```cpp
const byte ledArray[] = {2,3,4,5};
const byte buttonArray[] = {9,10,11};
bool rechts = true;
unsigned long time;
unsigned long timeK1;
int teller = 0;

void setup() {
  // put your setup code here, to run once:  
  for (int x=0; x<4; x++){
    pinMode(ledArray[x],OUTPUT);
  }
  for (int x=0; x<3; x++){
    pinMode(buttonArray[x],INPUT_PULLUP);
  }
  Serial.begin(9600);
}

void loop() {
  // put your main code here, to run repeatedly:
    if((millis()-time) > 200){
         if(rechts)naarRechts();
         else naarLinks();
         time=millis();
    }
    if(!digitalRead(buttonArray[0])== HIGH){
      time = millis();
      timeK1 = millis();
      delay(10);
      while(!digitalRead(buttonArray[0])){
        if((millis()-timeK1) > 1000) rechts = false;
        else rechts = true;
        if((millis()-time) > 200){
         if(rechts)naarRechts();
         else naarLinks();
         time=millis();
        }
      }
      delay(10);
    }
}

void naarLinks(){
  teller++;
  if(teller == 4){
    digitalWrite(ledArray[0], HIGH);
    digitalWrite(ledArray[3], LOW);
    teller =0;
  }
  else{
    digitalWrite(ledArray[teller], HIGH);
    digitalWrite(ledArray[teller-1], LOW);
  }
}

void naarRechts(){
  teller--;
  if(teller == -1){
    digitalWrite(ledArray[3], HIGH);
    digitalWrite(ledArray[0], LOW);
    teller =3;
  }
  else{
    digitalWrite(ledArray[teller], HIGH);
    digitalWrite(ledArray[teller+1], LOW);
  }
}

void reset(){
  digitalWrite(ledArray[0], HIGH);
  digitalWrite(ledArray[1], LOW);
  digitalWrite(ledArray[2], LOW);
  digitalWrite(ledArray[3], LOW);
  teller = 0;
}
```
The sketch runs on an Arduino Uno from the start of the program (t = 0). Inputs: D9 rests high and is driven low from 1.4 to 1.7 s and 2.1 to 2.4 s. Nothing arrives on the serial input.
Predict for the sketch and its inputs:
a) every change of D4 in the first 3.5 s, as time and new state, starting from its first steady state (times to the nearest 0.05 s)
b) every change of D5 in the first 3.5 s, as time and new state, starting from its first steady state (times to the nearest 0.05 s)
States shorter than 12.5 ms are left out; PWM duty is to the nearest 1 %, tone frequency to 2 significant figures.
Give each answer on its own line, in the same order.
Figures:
0 s low; 0.4 s high; 0.6 s low; 1.2 s high; 1.6 s low; 2.3 s high; 2.5 s low; 3.1 s high; 3.3 s low
0 s low; 0.2 s high; 0.4 s low; 1 s high; 1.2 s low; 2 s high; 2.3 s low; 2.9 s high; 3.1 s low
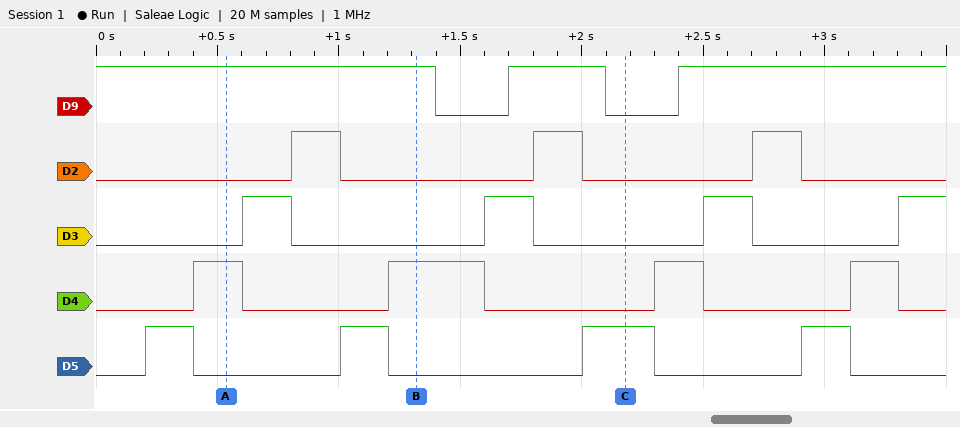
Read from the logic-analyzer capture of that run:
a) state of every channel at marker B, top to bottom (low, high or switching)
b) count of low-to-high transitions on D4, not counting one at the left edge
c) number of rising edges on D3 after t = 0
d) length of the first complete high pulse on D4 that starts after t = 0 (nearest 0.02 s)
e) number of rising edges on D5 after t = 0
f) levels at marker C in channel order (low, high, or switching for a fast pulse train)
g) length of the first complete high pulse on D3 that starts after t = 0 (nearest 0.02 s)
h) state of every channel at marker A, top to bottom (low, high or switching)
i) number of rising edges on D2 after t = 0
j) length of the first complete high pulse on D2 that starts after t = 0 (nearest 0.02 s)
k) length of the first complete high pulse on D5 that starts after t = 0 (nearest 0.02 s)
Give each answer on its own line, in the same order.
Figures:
D9 high, D2 low, D3 low, D4 high, D5 low
4
4
0.20 s
4
D9 low, D2 low, D3 low, D4 low, D5 high
0.20 s
D9 high, D2 low, D3 low, D4 high, D5 low
3
0.20 s
0.20 s
